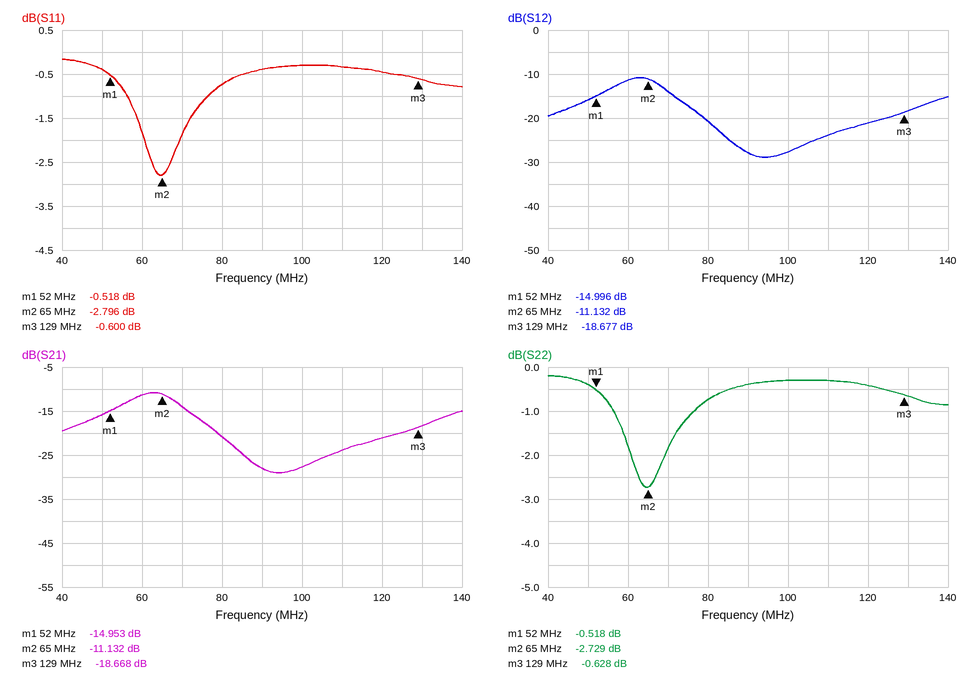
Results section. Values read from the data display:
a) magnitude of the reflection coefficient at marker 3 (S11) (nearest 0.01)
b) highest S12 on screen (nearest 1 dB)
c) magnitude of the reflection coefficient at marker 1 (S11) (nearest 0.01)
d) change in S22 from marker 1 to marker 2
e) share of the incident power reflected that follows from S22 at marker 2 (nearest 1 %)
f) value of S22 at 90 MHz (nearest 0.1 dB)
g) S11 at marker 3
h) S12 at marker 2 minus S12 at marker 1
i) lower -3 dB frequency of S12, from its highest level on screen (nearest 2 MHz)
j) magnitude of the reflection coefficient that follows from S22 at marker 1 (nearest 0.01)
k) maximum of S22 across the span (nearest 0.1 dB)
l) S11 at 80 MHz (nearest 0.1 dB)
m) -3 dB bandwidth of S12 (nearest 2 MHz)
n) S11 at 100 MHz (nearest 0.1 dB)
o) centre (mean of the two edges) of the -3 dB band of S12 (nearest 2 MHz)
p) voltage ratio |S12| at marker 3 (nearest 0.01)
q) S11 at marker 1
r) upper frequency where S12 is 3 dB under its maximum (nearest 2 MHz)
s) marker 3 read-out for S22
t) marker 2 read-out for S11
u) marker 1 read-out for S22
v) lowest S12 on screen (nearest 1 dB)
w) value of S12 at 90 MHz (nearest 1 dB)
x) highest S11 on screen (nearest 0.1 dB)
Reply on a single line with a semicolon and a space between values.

0.93; -11 dB; 0.94; -2.211 dB; 53 %; -0.4 dB; -0.600 dB; 3.864 dB; 54 MHz; 0.94; -0.2 dB; -0.7 dB; 16 MHz; -0.3 dB; 62 MHz; 0.12; -0.518 dB; 70 MHz; -0.628 dB; -2.796 dB; -0.518 dB; -29 dB; -28 dB; -0.2 dB
